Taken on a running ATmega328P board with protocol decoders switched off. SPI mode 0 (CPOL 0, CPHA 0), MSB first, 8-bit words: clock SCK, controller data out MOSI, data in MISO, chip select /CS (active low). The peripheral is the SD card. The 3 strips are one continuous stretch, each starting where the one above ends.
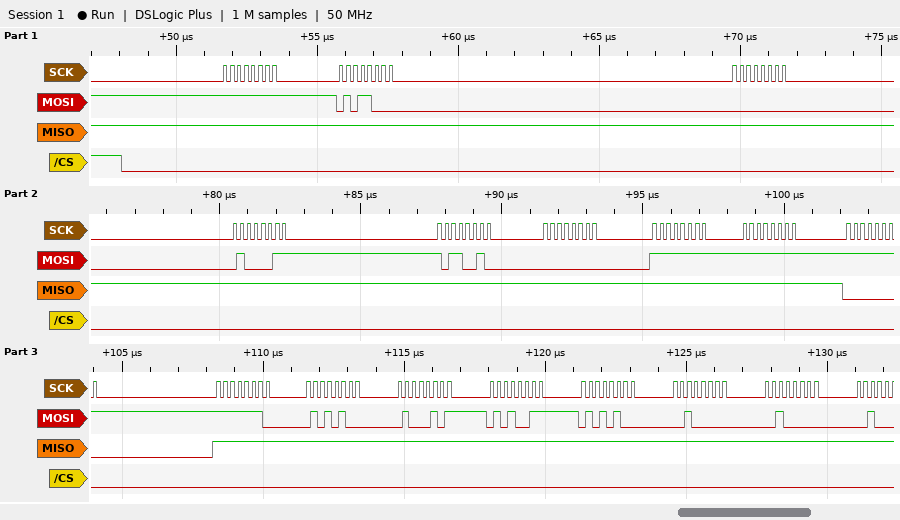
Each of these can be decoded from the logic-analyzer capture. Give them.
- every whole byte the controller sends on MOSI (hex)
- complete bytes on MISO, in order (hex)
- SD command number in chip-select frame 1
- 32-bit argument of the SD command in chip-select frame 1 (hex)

FF 58 00 43 B2 00 FF FF FF FE 54 45 53 54 20 20
FF FF FF FF FF FF FF FF 00 FF FF FF FF FF FF FF
CMD24
0x0043B200
